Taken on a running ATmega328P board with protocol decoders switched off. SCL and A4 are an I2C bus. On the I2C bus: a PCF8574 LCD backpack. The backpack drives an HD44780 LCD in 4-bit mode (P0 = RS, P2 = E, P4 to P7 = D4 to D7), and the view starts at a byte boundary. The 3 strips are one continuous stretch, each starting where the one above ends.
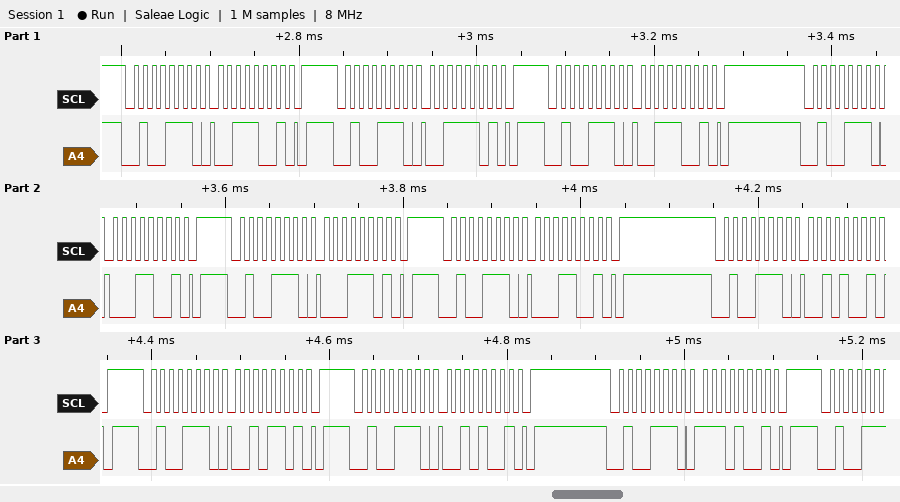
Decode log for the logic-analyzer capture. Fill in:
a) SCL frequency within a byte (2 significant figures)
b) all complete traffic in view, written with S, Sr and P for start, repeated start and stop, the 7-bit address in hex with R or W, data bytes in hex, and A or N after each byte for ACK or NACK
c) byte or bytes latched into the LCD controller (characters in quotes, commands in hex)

100 kHz
S 27W A 39 A P S 27W A 3D A P S 27W A 39 A P S 27W A 19 A P S 27W A 1D A P S 27W A 19 A P S 27W A 29 A P S 27W A 2D A P S 27W A 29 A P S 27W A E9 A P
'1'
